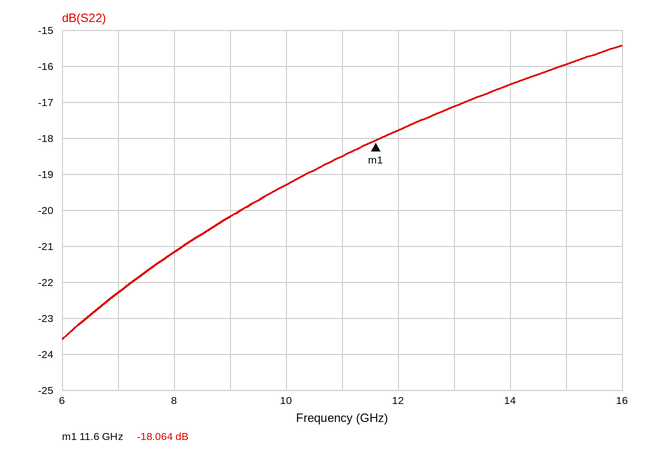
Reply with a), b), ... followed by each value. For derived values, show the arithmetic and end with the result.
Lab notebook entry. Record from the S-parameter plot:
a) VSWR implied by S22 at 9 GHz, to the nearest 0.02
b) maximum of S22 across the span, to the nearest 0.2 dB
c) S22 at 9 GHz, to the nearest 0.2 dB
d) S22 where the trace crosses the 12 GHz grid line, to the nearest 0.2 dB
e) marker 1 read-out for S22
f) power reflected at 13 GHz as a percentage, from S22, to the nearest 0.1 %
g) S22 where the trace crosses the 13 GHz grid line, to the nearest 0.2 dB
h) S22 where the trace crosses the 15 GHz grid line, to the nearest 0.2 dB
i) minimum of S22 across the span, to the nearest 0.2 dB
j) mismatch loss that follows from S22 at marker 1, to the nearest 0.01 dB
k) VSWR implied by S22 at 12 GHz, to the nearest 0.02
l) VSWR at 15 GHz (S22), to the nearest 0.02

a) |Γ| = 10^(-20.2/20) = 0.0977; VSWR = (1 + 0.0977)/(1 − 0.0977) ≈ 1.22
b) -15.4 dB
c) -20.2 dB
d) -17.8 dB
e) -18.064 dB
f) 10^(-17.2/10) ≈ 1.9 %
g) -17.2 dB
h) -16.0 dB
i) -23.6 dB
j) −10 log10(1 − 10^(-18.064/10)) ≈ 0.07 dB
k) |Γ| = 10^(-17.8/20) = 0.1288; VSWR = (1 + 0.1288)/(1 − 0.1288) ≈ 1.30
l) |Γ| = 10^(-16/20) = 0.1585; VSWR = (1 + 0.1585)/(1 − 0.1585) ≈ 1.38
